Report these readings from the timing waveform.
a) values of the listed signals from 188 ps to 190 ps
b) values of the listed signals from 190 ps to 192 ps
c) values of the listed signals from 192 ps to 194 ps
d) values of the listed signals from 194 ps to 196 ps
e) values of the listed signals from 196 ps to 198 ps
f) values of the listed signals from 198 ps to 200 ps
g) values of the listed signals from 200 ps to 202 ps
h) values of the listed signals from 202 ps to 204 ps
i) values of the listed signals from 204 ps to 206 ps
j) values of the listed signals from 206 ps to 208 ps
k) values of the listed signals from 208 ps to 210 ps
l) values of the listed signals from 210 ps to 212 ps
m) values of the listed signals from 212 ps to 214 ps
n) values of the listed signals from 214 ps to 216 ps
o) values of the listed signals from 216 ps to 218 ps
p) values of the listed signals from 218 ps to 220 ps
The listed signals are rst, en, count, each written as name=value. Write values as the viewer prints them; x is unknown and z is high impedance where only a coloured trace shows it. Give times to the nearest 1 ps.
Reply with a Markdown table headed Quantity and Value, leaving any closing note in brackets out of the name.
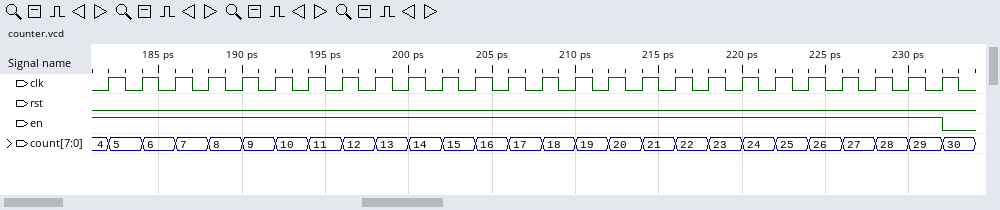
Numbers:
| Quantity | Value |
|---|---|
| values of the listed signals from 188 ps to 190 ps | rst=0, en=1, count=8 |
| values of the listed signals from 190 ps to 192 ps | rst=0, en=1, count=9 |
| values of the listed signals from 192 ps to 194 ps | rst=0, en=1, count=10 |
| values of the listed signals from 194 ps to 196 ps | rst=0, en=1, count=11 |
| values of the listed signals from 196 ps to 198 ps | rst=0, en=1, count=12 |
| values of the listed signals from 198 ps to 200 ps | rst=0, en=1, count=13 |
| values of the listed signals from 200 ps to 202 ps | rst=0, en=1, count=14 |
| values of the listed signals from 202 ps to 204 ps | rst=0, en=1, count=15 |
| values of the listed signals from 204 ps to 206 ps | rst=0, en=1, count=16 |
| values of the listed signals from 206 ps to 208 ps | rst=0, en=1, count=17 |
| values of the listed signals from 208 ps to 210 ps | rst=0, en=1, count=18 |
| values of the listed signals from 210 ps to 212 ps | rst=0, en=1, count=19 |
| values of the listed signals from 212 ps to 214 ps | rst=0, en=1, count=20 |
| values of the listed signals from 214 ps to 216 ps | rst=0, en=1, count=21 |
| values of the listed signals from 216 ps to 218 ps | rst=0, en=1, count=22 |
| values of the listed signals from 218 ps to 220 ps | rst=0, en=1, count=23 |
